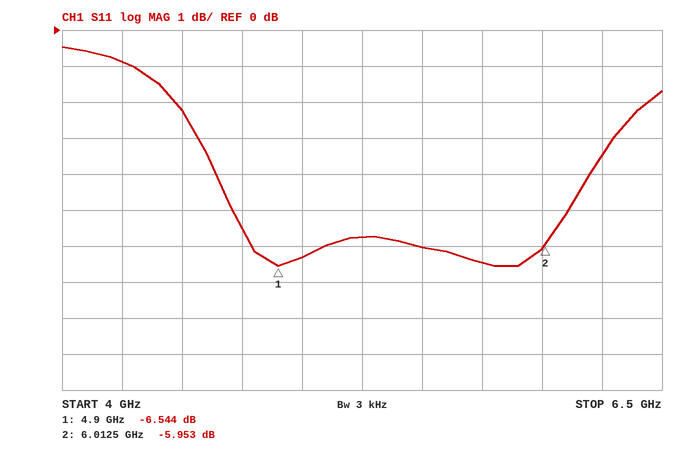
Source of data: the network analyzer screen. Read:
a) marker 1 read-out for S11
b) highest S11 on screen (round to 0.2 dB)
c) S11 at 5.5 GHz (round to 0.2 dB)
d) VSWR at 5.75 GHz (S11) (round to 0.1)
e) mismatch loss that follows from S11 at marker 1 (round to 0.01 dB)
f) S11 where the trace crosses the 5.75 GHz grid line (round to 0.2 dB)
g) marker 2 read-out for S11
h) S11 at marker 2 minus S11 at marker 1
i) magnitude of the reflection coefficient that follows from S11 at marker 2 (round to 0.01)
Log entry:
-6.544 dB
-0.4 dB
-6.0 dB
2.8
1.09 dB
-6.4 dB
-5.953 dB
0.591 dB
0.50
